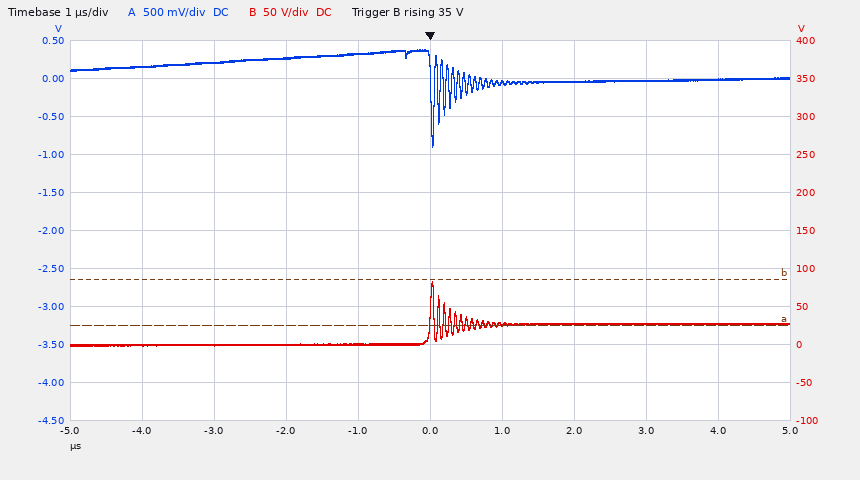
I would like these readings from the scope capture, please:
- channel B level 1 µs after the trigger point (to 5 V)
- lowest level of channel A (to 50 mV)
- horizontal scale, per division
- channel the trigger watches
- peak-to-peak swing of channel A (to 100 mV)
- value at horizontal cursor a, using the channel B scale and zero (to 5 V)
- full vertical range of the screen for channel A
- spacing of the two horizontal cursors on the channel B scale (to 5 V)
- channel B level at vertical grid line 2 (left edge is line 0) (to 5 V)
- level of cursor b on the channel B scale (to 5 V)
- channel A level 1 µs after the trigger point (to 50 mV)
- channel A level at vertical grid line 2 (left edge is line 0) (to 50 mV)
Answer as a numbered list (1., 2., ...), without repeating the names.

1. 25 V
2. -900 mV
3. 1 µs
4. channel B
5. 1.30 V
6. 25 V
7. 5 V
8. 60 V
9. 0 V
10. 85 V
11. -50 mV
12. 200 mV
